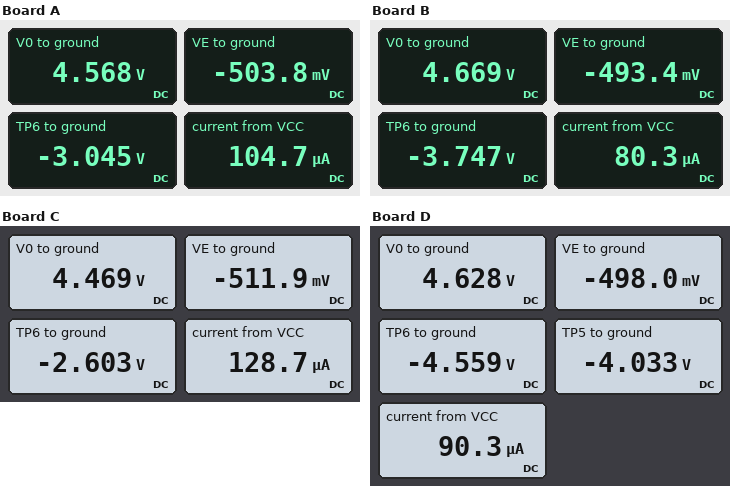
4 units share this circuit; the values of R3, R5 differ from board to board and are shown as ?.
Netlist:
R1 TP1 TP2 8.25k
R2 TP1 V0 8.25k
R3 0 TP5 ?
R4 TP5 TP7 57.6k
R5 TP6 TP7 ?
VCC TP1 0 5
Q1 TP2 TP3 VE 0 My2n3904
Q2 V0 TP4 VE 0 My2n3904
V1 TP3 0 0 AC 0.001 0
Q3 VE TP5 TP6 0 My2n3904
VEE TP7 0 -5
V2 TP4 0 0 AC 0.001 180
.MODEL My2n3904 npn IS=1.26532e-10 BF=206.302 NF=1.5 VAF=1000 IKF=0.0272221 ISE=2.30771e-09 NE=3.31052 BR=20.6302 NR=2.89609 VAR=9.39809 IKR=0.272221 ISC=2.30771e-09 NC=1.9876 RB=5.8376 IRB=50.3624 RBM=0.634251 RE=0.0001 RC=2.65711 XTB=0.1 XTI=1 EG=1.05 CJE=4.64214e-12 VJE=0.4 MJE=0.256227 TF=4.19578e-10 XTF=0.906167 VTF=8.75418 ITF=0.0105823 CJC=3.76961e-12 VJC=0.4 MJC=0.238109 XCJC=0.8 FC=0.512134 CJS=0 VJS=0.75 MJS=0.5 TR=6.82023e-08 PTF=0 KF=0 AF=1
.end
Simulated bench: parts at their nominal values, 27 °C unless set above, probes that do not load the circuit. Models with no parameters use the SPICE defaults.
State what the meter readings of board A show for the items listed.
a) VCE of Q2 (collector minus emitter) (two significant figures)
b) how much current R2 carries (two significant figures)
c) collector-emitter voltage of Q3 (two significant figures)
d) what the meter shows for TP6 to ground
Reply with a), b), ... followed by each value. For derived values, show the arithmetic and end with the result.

a) 4.568 V - (-503.8 mV) = 5.1 V
b) (5 V - 4.568 V) / 8.25 kΩ = 52 µA
c) -503.8 mV - (-3.045 V) = 2.5 V
d) -3.045 V
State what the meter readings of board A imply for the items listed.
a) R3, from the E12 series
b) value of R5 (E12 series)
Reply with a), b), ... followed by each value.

a) 56 kΩ
b) 18 kΩ
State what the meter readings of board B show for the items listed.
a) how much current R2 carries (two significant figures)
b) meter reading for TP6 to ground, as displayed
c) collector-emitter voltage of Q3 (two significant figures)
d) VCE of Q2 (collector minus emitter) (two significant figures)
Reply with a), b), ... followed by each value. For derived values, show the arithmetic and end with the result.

a) (5 V - 4.669 V) / 8.25 kΩ = 40 µA
b) -3.747 V
c) -493.4 mV - (-3.747 V) = 3.3 V
d) 4.669 V - (-493.4 mV) = 5.2 V
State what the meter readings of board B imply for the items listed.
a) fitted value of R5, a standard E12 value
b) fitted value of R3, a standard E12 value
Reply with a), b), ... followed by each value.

a) 15 kΩ
b) 100 kΩ
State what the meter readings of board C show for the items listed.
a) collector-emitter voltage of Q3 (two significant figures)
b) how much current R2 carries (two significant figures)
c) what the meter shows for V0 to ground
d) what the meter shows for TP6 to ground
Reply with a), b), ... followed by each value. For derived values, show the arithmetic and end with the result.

a) -511.9 mV - (-2.603 V) = 2.1 V
b) (5 V - 4.469 V) / 8.25 kΩ = 64 µA
c) 4.469 V
d) -2.603 V
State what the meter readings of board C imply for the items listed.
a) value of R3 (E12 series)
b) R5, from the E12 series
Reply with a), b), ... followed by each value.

a) 39 kΩ
b) 18 kΩ
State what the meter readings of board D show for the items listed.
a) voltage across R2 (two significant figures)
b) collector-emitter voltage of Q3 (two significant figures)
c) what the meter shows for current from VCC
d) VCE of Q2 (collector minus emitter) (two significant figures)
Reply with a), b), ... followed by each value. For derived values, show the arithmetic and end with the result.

a) 5 V - 4.628 V = 370 mV
b) -498 mV - (-4.559 V) = 4.1 V
c) 90.3 µA
d) 4.628 V - (-498 mV) = 5.1 V
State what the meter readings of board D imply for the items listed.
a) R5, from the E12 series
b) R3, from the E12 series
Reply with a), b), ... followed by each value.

a) 4.7 kΩ
b) 220 kΩ
